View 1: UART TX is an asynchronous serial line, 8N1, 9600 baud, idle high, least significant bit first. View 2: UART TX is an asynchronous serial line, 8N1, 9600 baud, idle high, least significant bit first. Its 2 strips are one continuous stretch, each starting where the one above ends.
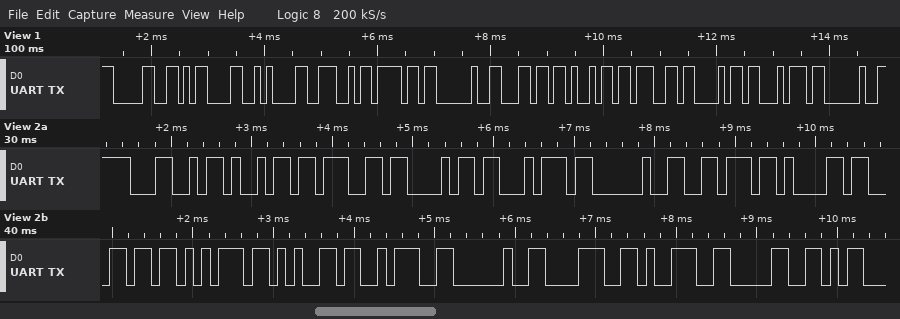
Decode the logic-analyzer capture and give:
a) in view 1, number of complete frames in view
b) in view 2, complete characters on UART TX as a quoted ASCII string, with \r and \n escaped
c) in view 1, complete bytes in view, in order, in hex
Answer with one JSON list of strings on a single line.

["12", "\"Light value: 890\"", "30 0D 0A 4E 6F 20 6C 69 67 68 74 20"]
